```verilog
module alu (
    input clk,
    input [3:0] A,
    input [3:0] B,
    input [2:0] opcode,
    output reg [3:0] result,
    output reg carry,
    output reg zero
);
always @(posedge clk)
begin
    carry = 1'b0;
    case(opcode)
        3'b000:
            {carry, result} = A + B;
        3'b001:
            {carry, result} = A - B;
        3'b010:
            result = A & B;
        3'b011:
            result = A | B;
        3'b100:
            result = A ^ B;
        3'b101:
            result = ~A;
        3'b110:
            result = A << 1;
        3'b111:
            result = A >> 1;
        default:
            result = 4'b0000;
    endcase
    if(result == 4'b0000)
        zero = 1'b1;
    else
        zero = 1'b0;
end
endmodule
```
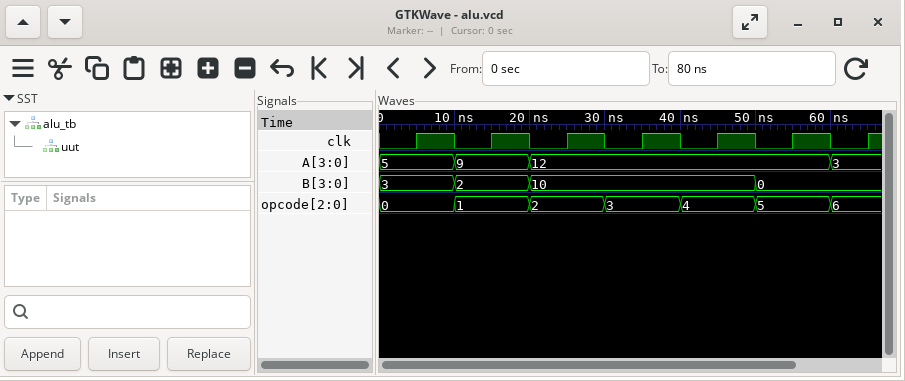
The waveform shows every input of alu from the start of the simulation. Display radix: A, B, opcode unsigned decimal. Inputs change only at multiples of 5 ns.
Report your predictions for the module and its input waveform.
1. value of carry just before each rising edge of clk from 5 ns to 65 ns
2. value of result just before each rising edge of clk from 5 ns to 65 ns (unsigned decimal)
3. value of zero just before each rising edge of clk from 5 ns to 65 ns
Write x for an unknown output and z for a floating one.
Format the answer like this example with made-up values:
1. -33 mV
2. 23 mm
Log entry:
1. x 0 0 0 0 0 0
2. x, 8, 7, 8, 14, 6, 3
3. x 0 0 0 0 0 0
